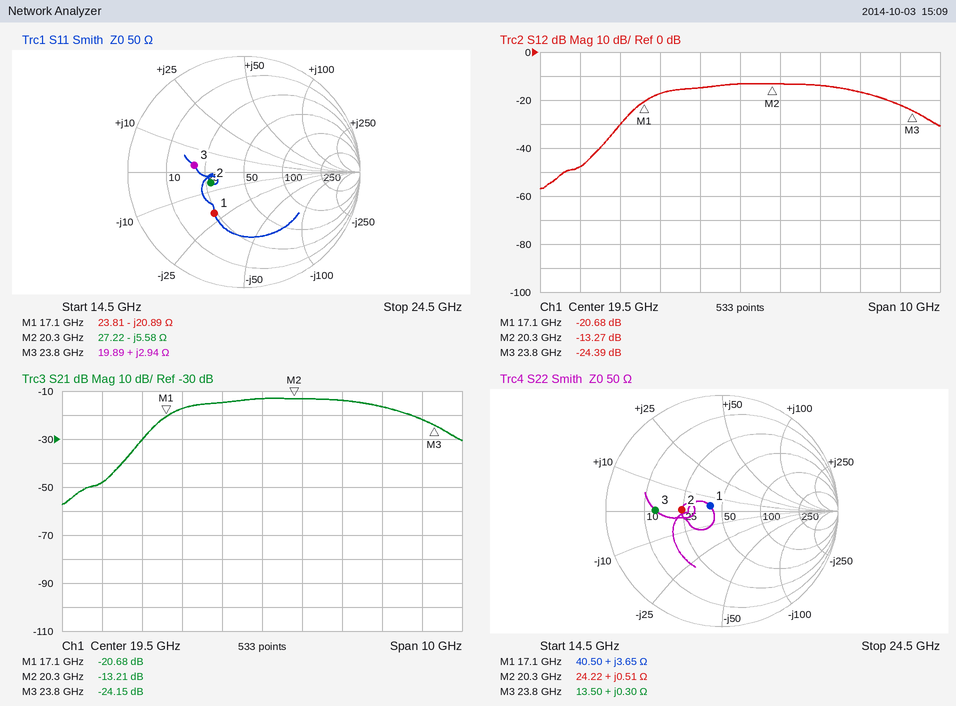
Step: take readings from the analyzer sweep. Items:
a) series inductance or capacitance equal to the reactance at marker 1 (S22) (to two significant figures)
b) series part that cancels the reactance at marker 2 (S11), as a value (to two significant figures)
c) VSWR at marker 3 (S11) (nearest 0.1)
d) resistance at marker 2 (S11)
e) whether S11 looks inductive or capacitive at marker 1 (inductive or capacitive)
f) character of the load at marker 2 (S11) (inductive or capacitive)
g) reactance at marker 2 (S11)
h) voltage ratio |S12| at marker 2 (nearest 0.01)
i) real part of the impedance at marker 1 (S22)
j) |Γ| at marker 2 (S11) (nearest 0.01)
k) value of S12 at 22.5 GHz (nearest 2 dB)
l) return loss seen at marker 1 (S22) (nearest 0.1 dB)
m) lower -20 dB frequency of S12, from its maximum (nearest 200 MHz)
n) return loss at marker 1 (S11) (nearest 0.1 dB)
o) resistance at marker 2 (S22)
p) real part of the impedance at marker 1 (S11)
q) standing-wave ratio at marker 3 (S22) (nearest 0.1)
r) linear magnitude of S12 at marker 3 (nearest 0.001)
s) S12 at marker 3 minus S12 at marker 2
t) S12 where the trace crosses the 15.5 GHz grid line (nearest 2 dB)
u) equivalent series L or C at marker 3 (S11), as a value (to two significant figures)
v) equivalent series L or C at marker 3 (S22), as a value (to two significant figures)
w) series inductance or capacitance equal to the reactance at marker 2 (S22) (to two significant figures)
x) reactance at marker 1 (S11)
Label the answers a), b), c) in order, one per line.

a) 34 pH
b) 44 pH
c) 2.5
d) 27.22 Ω
e) capacitive
f) capacitive
g) -5.58 Ω
h) 0.22
i) 40.50 Ω
j) 0.30
k) -16 dB
l) 19.0 dB
m) 16.4 GHz
n) 7.2 dB
o) 24.22 Ω
p) 23.81 Ω
q) 3.7
r) 0.060
s) -11.12 dB
t) -48 dB
u) 20 pH
v) 2.0 pH
w) 4.0 pH
x) -20.89 Ω
